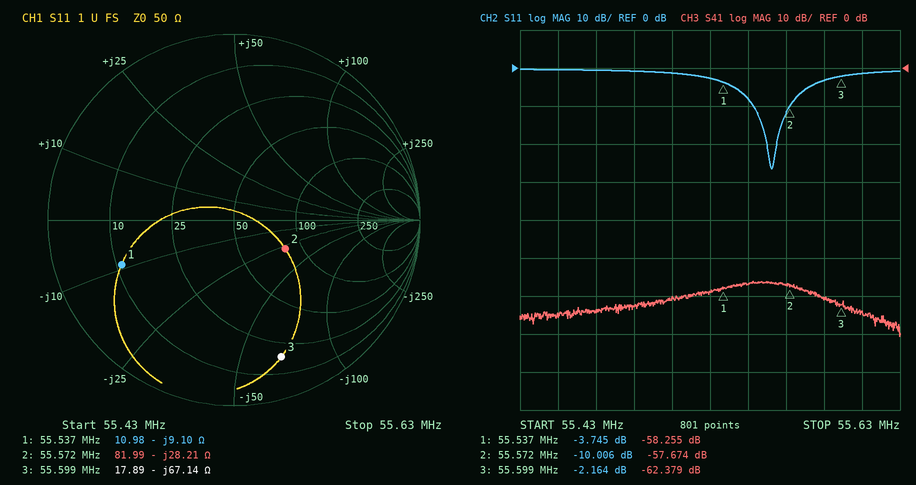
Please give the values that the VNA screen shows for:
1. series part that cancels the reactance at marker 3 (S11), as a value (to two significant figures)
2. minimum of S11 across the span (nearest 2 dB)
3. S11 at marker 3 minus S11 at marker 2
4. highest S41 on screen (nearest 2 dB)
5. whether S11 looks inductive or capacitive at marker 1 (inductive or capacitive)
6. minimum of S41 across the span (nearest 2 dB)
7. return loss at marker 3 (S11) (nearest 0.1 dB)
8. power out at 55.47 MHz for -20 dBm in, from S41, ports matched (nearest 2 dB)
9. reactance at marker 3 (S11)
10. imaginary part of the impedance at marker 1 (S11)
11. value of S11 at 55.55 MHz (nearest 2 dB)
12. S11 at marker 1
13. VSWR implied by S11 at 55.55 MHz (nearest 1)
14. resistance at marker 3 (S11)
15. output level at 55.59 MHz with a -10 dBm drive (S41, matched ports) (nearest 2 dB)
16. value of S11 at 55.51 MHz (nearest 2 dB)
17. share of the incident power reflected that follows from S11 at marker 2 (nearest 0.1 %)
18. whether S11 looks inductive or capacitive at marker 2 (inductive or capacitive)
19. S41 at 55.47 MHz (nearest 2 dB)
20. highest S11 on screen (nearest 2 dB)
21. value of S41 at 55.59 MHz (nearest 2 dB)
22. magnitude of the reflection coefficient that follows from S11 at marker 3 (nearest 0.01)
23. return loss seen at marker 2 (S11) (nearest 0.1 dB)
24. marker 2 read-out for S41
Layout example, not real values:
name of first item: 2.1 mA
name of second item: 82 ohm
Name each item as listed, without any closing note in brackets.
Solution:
series part that cancels the reactance at marker 3 (S11), as a value: 190 nH
minimum of S11 across the span: -26 dB
S11 at marker 3 minus S11 at marker 2: 7.842 dB
highest S41 on screen: -56 dB
whether S11 looks inductive or capacitive at marker 1: capacitive
minimum of S41 across the span: -70 dB
return loss at marker 3 (S11): 2.2 dB
power out at 55.47 MHz for -20 dBm in, from S41, ports matched: -84 dBm
reactance at marker 3: -67.14 Ω
imaginary part of the impedance at marker 1: -9.10 Ω
value of S11 at 55.55 MHz: -8 dB
S11 at marker 1: -3.745 dB
VSWR implied by S11 at 55.55 MHz: 2
resistance at marker 3: 17.89 Ω
output level at 55.59 MHz with a -10 dBm drive (S41, matched ports): -70 dBm
value of S11 at 55.51 MHz: -2 dB
share of the incident power reflected that follows from S11 at marker 2: 10.0 %
whether S11 looks inductive or capacitive at marker 2: capacitive
S41 at 55.47 MHz: -64 dB
highest S11 on screen: 0 dB
value of S41 at 55.59 MHz: -60 dB
magnitude of the reflection coefficient that follows from S11 at marker 3: 0.78
return loss seen at marker 2 (S11): 10.0 dB
marker 2 read-out for S41: -57.674 dB
